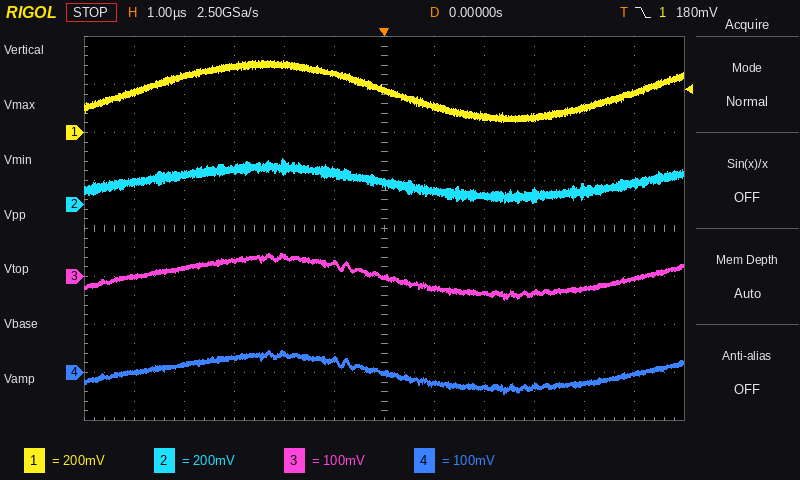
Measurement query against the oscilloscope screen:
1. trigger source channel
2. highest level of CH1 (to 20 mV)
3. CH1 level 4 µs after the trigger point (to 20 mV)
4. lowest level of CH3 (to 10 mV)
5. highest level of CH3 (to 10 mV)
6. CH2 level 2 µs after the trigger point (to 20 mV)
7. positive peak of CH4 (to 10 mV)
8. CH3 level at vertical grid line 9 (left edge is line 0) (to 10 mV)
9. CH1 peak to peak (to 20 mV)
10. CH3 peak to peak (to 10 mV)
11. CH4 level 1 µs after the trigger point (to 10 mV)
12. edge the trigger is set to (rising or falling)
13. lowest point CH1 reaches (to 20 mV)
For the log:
CH1
300 mV
100 mV
-50 mV
50 mV
40 mV
50 mV
-30 mV
260 mV
100 mV
-20 mV
falling
40 mV
